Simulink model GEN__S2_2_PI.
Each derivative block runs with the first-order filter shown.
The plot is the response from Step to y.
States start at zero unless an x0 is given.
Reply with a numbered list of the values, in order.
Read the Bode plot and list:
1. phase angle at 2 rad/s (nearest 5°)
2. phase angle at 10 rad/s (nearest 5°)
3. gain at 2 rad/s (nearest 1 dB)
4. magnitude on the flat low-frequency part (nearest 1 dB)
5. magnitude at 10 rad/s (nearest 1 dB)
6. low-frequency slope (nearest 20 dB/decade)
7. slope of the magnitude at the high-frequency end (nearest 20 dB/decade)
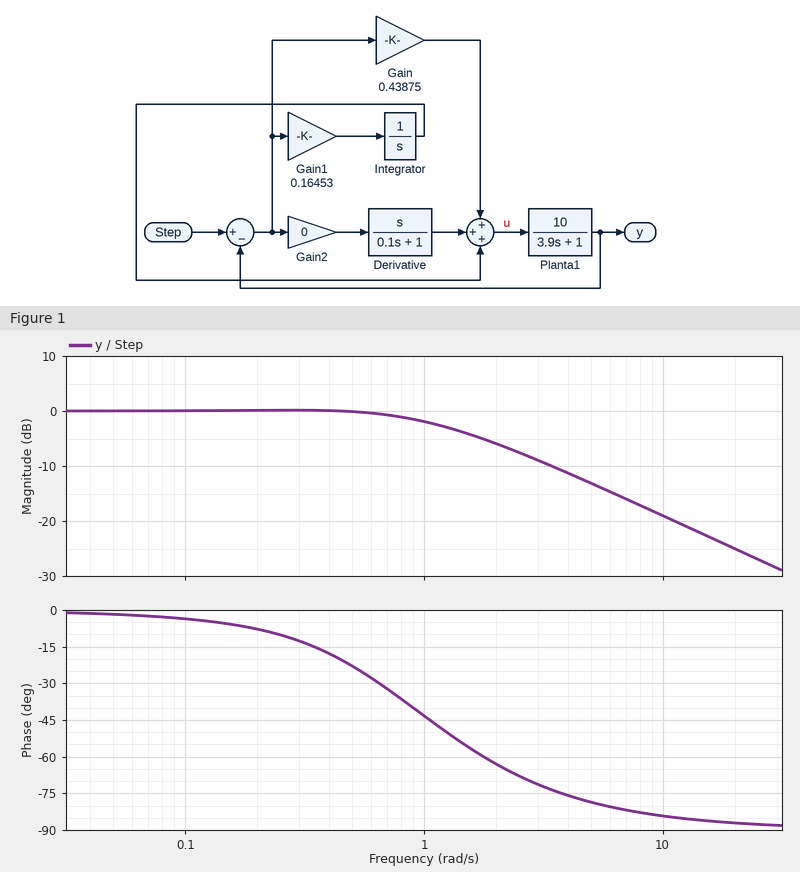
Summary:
1. -65°
2. -85°
3. -6 dB
4. 0 dB
5. -19 dB
6. 0 dB/decade
7. -20 dB/decade
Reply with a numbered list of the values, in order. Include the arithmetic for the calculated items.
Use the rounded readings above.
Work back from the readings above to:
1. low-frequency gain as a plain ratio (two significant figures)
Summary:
1. 10^(0 / 20) = 1.0
